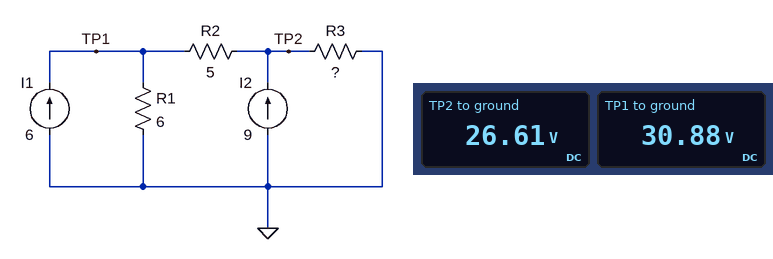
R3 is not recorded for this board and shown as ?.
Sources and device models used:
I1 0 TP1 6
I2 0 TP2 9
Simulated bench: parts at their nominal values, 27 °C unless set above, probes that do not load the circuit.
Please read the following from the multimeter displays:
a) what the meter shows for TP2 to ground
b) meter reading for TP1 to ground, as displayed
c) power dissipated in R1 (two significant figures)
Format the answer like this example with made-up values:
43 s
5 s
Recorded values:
26.61 V
30.88 V
160 W
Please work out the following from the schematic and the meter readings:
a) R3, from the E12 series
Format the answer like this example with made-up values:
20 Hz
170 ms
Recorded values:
2.7 Ω
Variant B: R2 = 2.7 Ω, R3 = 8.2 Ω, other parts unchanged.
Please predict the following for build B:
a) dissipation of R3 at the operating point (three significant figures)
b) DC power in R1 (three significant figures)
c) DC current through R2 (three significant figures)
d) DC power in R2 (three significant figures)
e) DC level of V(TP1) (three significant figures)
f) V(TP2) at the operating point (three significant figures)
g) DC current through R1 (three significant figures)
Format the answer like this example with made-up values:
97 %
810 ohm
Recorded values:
375 W
407 W
2.24 A
13.5 W
49.4 V
55.5 V
8.24 A
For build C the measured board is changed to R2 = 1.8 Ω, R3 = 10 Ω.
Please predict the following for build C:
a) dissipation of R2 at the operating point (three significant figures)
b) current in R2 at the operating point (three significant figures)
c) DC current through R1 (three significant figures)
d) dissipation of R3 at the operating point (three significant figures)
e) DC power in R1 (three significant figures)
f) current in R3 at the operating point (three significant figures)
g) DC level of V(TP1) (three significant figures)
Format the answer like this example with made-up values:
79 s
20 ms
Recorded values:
16.6 W
3.03 A
9.03 A
356 W
490 W
5.97 A
54.2 V
